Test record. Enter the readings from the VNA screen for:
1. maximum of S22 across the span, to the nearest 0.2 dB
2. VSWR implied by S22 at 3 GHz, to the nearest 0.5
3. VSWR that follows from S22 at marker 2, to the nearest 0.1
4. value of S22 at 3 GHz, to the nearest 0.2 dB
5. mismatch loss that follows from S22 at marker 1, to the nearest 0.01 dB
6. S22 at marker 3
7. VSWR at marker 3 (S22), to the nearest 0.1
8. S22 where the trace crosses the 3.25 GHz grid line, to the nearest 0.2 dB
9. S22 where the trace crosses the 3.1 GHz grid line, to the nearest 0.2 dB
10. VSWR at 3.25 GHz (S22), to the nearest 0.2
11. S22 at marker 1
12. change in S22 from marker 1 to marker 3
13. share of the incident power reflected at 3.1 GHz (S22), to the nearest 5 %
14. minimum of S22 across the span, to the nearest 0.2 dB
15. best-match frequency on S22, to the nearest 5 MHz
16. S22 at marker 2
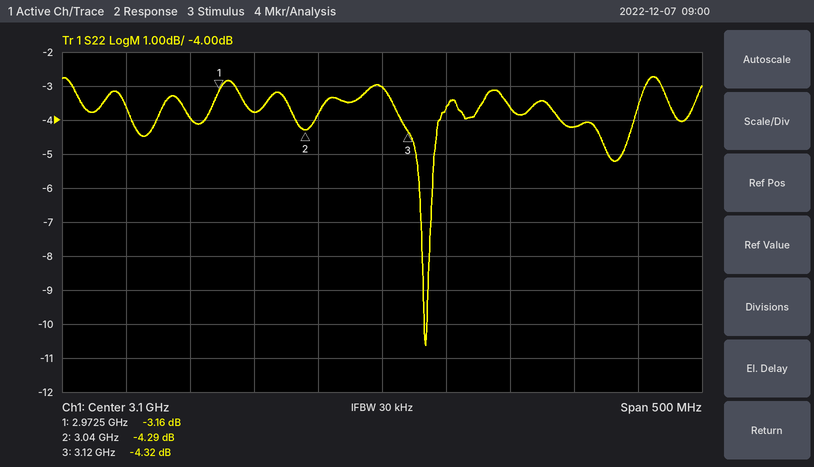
-2.8 dB
4.5
4.1
-3.8 dB
2.87 dB
-4.32 dB
4.1
-4.2 dB
-3.0 dB
4.2
-3.16 dB
-1.16 dB
50 %
-10.6 dB
3.135 GHz
-4.29 dB
